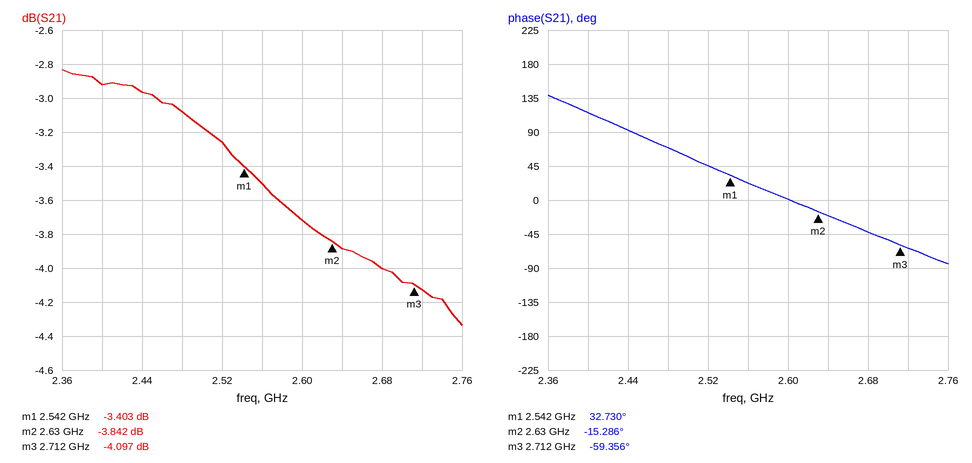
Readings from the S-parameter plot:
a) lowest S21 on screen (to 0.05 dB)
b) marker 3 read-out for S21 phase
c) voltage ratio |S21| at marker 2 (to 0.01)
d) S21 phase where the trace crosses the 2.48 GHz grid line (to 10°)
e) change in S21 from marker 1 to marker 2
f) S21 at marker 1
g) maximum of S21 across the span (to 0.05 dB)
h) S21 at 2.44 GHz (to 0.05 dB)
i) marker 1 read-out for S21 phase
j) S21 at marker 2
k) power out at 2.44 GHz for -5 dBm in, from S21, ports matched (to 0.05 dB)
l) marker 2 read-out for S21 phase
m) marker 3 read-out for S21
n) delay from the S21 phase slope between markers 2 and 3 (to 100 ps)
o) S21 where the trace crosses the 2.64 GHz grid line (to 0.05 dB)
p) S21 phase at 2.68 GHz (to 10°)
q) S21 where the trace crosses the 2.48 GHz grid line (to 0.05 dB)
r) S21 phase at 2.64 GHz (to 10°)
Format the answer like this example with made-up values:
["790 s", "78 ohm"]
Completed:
["-4.35 dB", "-59.356°", "0.64", "70°", "-0.439 dB", "-3.403 dB", "-2.85 dB", "-2.95 dB", "32.730°", "-3.842 dB", "-7.95 dBm", "-15.286°", "-4.097 dB", "1.5 ns", "-3.90 dB", "-40°", "-3.10 dB", "-20°"]
